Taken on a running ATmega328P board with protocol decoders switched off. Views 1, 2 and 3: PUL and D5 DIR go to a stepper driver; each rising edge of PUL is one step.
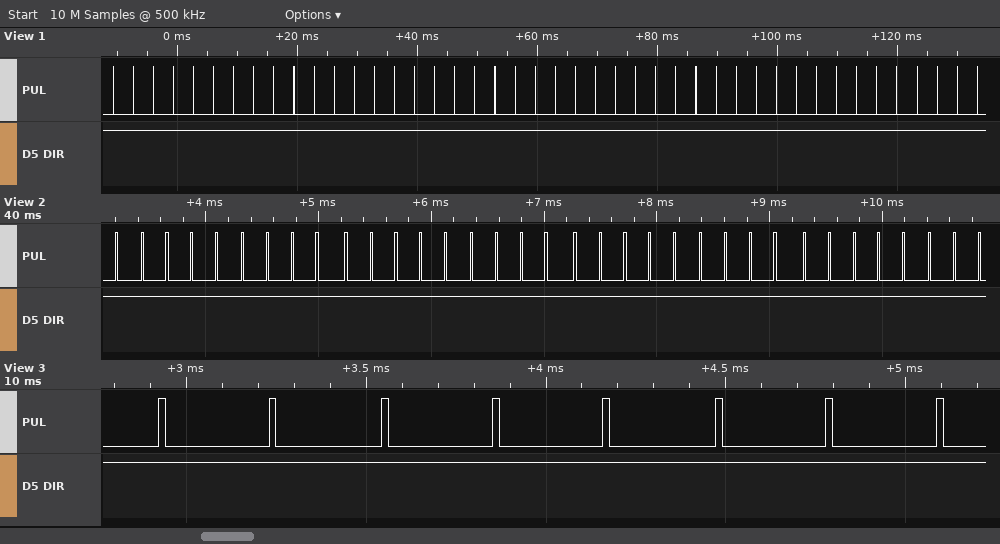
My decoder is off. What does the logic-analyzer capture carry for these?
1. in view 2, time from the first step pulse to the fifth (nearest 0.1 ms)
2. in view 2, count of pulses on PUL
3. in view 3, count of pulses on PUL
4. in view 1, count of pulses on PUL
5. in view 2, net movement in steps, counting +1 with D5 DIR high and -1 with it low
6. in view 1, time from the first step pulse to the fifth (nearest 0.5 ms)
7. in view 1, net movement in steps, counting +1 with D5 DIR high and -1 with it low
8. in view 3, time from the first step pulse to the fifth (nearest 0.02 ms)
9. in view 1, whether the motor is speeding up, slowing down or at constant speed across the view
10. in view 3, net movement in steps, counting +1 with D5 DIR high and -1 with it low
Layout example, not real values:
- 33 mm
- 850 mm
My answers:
- 0.9 ms
- 35
- 8
- 44
- +35
- 13.5 ms
- +44
- 1.24 ms
- constant speed
- +8
